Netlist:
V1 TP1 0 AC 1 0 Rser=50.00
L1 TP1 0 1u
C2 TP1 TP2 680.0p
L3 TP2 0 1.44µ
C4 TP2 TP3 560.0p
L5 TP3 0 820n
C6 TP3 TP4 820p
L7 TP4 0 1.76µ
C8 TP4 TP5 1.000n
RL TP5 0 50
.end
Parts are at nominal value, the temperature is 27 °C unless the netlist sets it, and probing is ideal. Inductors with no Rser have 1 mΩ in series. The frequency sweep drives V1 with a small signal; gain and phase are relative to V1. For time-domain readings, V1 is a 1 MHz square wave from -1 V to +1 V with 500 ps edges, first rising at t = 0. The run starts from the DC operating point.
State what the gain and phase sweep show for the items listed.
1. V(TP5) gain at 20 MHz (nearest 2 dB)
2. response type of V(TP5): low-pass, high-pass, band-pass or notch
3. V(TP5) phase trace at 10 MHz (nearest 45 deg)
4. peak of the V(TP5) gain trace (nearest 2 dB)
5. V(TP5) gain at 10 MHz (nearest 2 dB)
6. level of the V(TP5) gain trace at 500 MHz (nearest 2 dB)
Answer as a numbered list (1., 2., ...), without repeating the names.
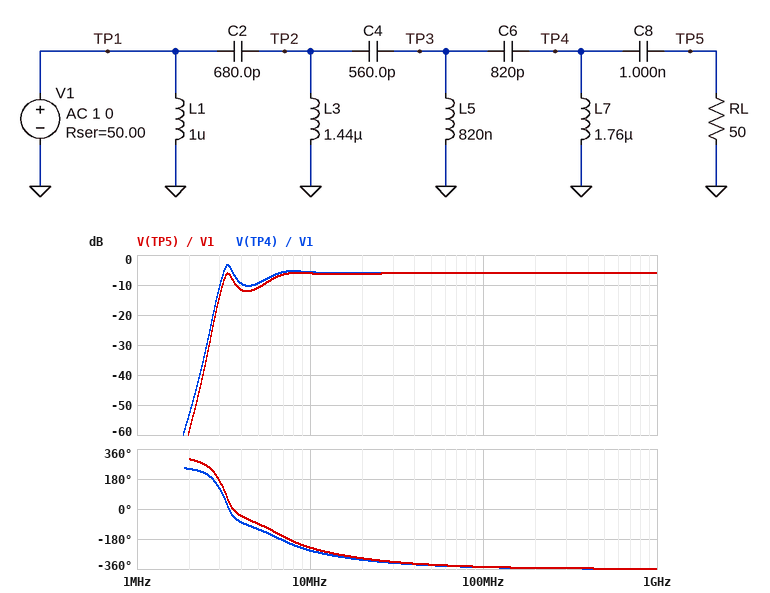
1. -6 dB
2. high-pass
3. -225 deg
4. -6 dB
5. -6 dB
6. -6 dB
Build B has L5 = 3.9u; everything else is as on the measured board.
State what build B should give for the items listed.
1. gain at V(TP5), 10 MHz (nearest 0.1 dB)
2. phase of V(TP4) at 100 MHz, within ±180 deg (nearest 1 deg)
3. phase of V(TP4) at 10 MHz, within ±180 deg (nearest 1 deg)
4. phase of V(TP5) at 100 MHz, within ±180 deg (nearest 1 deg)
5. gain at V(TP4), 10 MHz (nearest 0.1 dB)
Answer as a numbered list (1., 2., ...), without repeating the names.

1. -6.7 dB
2. 9 deg
3. 91 deg
4. 11 deg
5. -6.3 dB
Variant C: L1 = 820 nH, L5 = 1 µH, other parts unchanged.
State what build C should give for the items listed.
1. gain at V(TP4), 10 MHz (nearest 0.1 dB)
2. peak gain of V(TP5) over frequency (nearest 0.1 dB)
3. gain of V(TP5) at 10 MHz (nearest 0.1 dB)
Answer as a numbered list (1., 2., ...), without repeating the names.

1. -5.9 dB
2. -6.0 dB
3. -6.3 dB
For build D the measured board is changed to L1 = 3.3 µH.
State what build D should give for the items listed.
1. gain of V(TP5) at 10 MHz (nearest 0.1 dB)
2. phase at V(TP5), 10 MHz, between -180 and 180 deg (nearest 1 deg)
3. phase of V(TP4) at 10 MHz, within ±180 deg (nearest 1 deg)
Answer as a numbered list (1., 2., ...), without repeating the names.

1. -6.3 dB
2. 115 deg
3. 97 deg
